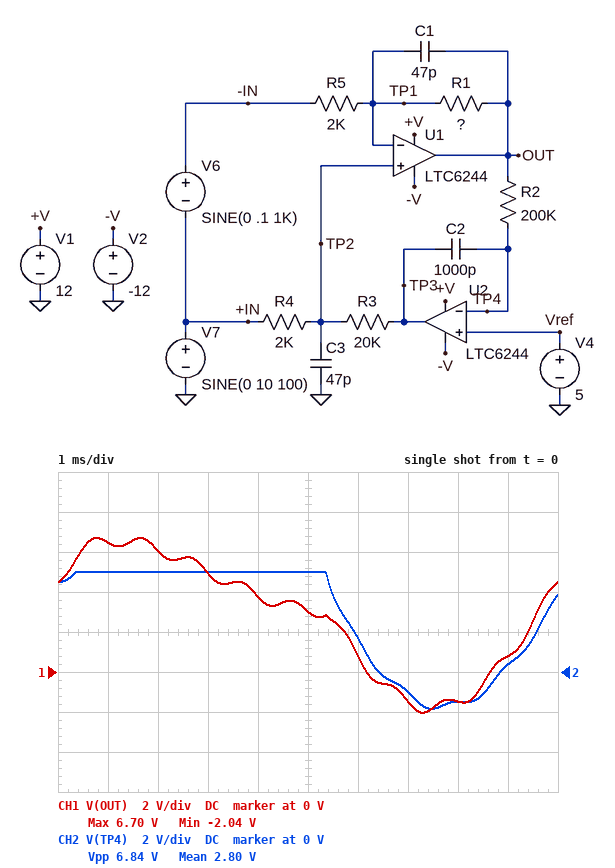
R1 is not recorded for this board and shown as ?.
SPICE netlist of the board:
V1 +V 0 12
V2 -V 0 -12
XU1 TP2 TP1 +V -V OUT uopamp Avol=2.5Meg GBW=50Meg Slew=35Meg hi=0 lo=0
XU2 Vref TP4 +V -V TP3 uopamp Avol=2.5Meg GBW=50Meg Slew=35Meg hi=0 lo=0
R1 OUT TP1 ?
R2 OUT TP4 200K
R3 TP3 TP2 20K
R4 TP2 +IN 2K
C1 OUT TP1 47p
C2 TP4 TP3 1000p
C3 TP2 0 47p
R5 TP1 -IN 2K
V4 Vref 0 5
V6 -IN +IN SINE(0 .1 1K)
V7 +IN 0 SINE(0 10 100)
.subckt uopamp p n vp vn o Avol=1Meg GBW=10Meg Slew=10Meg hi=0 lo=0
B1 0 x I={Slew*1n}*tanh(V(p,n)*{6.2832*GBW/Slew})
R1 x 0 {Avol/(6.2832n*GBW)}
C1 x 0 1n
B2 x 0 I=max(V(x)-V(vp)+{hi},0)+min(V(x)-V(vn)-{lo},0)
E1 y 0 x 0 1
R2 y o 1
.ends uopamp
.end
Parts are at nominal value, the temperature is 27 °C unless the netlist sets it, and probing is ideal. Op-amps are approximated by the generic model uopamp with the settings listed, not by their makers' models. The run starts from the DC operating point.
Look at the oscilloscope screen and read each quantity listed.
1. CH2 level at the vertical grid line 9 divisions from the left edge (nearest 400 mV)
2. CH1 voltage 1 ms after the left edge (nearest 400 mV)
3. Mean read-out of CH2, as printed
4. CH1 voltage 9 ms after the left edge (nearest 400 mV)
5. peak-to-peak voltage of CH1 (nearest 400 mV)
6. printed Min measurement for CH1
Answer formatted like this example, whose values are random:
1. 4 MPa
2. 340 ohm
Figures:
1. 400 mV
2. 6.4 V
3. 2.80 V
4. 800 mV
5. 8.8 V
6. -2.04 V
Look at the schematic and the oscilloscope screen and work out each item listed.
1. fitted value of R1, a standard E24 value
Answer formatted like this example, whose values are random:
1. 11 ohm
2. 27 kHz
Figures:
1. 6.2 kΩ
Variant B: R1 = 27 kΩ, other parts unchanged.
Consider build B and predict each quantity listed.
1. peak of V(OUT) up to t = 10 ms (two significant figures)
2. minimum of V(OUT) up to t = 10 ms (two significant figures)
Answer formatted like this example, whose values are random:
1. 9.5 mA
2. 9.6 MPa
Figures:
1. 6.2 V
2. 3.8 V
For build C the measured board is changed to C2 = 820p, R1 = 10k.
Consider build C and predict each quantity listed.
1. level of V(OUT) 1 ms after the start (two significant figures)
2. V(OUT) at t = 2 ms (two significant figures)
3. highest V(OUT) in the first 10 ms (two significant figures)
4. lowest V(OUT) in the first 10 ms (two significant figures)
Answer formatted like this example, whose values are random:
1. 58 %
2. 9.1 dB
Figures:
1. 5.5 V
2. 5.2 V
3. 6.2 V
4. 1.6 V
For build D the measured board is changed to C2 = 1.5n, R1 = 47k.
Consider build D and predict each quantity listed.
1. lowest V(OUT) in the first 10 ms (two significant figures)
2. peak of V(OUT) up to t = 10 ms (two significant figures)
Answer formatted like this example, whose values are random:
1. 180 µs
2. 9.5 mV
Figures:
1. 2.6 V
2. 7.5 V
